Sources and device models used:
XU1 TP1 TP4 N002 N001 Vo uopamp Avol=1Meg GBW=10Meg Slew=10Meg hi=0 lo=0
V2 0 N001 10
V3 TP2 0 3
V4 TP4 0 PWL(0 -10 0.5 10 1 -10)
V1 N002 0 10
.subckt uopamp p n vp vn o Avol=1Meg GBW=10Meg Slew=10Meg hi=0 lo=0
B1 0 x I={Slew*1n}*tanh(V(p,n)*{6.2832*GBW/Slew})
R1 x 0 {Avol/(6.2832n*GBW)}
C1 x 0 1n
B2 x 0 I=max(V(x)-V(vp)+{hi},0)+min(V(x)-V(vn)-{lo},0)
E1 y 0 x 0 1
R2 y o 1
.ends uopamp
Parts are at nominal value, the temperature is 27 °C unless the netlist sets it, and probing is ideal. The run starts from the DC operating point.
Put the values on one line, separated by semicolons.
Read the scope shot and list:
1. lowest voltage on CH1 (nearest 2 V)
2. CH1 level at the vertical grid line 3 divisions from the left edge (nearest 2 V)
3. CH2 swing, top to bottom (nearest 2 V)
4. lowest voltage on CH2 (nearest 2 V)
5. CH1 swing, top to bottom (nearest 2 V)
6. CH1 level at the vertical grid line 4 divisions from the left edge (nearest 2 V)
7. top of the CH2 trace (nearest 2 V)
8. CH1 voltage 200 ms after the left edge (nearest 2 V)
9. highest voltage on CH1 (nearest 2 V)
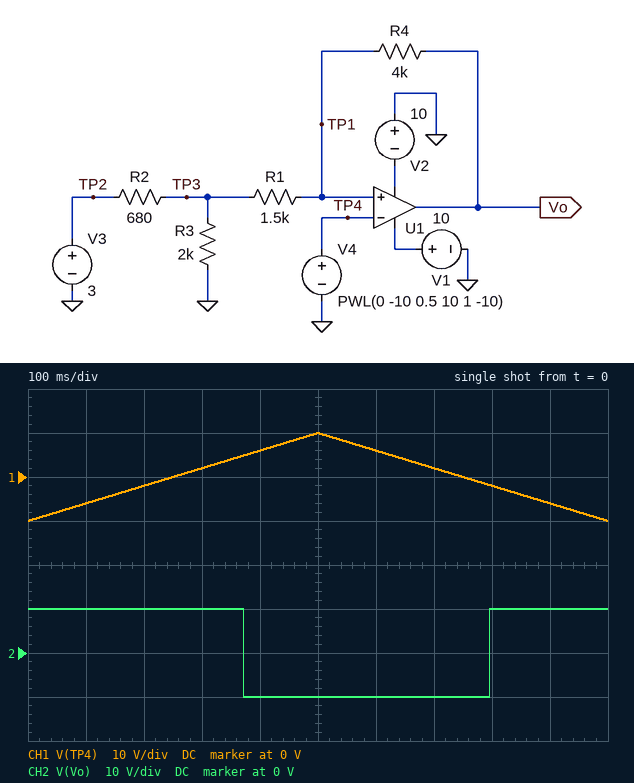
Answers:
-10 V; 2 V; 20 V; -10 V; 20 V; 6 V; 10 V; -2 V; 10 V
